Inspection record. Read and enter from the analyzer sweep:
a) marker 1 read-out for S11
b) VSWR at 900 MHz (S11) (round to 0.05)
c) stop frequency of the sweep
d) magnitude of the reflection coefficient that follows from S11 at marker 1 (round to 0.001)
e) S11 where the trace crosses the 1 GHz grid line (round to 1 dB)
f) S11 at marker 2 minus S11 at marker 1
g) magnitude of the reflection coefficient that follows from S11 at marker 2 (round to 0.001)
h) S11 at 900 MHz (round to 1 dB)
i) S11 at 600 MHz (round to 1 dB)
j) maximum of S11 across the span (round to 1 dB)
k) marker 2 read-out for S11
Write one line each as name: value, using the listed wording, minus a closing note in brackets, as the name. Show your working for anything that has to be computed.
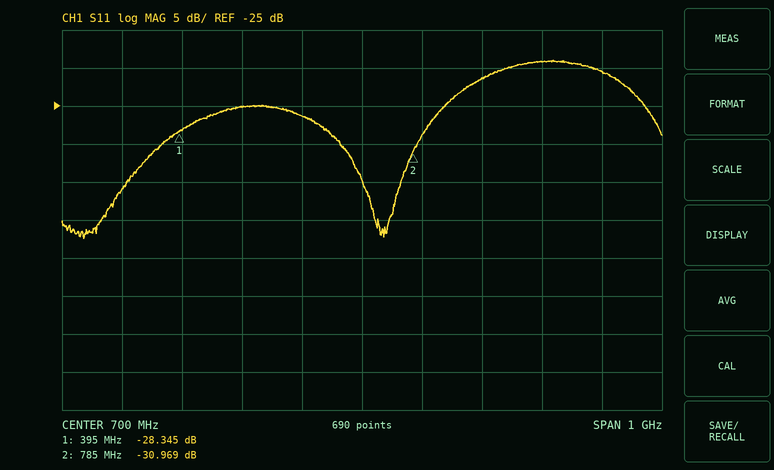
marker 1 read-out for S11: -28.345 dB
VSWR at 900 MHz (S11): |Γ| = 10^(-21/20) = 0.0891; VSWR = (1 + 0.0891)/(1 − 0.0891) ≈ 1.20
stop frequency of the sweep: 1.2 GHz
magnitude of the reflection coefficient that follows from S11 at marker 1: 10^(-28.345/20) ≈ 0.038
S11 where the trace crosses the 1 GHz grid line: -19 dB
S11 at marker 2 minus S11 at marker 1: -30.969 − (-28.345) = -2.624 dB
magnitude of the reflection coefficient that follows from S11 at marker 2: 10^(-30.969/20) ≈ 0.028
S11 at 900 MHz: -21 dB
S11 at 600 MHz: -26 dB
maximum of S11 across the span: -19 dB
marker 2 read-out for S11: -30.969 dB
